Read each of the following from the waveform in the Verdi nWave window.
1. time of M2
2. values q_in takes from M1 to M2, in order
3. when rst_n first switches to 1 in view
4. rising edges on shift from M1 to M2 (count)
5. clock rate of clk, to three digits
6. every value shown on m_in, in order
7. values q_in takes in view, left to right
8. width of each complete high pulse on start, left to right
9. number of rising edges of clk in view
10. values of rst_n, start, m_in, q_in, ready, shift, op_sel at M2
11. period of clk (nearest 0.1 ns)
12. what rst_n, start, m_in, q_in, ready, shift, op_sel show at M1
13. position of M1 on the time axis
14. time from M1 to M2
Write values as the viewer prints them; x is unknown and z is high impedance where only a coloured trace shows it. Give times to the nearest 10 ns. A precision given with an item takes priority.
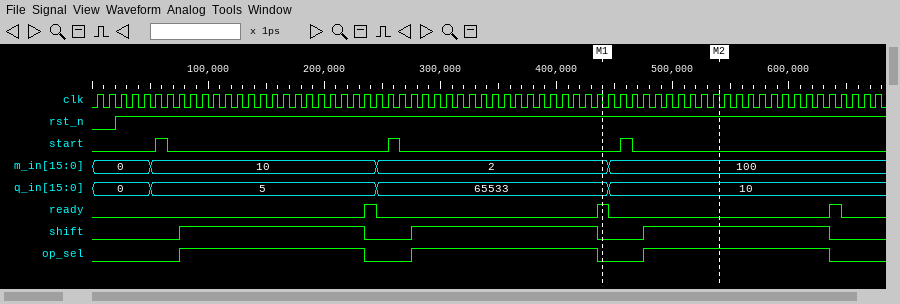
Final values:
540 ns
65533, 10
20 ns
1
100 MHz
0, 10, 2, 100
0, 5, 65533, 10
10 ns, 10 ns, 10 ns
68
rst_n=1, start=0, m_in=100, q_in=10, ready=0, shift=1, op_sel=1
10 ns
rst_n=1, start=0, m_in=2, q_in=65533, ready=1, shift=0, op_sel=0
440 ns
100 ns
